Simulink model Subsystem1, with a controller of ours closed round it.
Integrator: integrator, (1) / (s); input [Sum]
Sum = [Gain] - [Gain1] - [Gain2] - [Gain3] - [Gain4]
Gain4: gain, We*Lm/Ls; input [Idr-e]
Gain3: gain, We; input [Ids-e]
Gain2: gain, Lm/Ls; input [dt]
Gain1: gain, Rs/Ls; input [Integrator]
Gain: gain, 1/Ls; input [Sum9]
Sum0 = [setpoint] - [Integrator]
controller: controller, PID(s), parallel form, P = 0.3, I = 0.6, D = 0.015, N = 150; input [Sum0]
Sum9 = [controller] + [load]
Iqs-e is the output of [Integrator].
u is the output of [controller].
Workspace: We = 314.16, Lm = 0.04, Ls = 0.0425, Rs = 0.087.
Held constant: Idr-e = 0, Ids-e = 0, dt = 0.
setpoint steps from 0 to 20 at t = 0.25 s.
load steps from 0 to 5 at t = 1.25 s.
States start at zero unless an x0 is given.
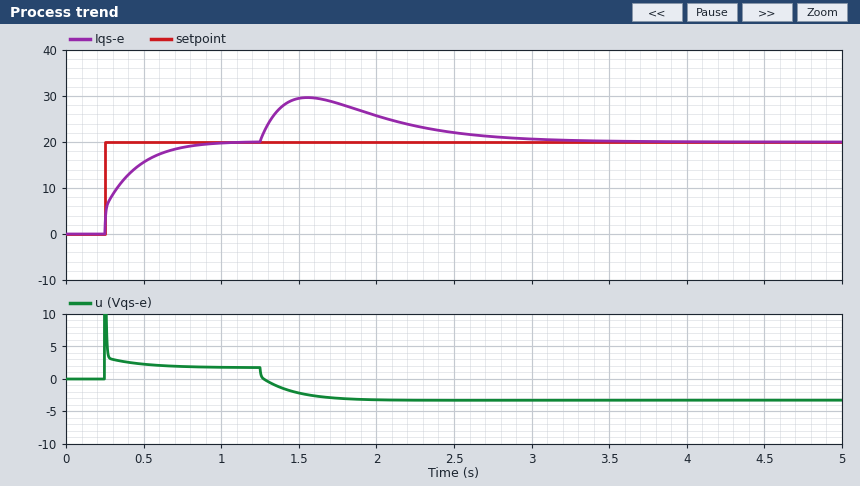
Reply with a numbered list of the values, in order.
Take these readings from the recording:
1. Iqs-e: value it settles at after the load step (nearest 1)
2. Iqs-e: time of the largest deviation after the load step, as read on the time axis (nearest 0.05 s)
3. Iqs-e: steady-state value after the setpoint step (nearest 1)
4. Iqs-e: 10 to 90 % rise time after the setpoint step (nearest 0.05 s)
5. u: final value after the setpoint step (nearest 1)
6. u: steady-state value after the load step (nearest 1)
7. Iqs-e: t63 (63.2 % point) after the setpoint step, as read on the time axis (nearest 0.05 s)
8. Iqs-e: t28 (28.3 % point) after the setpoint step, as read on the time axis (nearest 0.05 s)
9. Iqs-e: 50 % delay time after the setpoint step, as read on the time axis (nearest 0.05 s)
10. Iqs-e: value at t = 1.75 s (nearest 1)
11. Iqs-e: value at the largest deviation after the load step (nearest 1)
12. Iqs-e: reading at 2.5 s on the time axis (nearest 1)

1. 20
2. 1.55 s
3. 20
4. 0.40 s
5. 2
6. -3
7. 0.40 s
8. 0.25 s
9. 0.35 s
10. 28
11. 30
12. 22
